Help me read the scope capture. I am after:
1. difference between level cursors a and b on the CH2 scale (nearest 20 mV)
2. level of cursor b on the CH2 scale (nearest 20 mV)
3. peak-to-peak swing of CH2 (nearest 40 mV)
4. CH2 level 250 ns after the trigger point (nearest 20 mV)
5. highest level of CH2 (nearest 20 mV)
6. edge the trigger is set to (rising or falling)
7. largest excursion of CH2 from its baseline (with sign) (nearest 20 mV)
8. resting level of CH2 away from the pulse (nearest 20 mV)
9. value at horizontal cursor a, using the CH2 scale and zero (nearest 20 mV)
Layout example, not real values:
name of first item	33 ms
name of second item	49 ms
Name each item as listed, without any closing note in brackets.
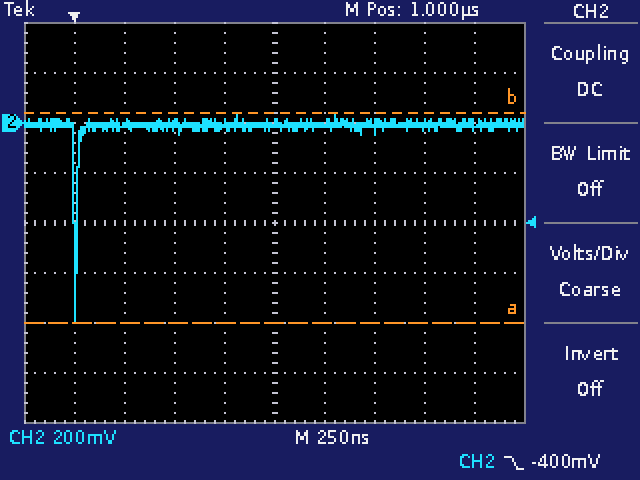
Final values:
difference between level cursors a and b on the CH2 scale	840 mV
level of cursor b on the CH2 scale	40 mV
peak-to-peak swing of CH2	840 mV
CH2 level 250 ns after the trigger point	0 mV
highest level of CH2	40 mV
edge the trigger is set to	falling
largest excursion of CH2 from its baseline (with sign)	-780 mV
resting level of CH2 away from the pulse	0 mV
value at horizontal cursor a, using the CH2 scale and zero	-800 mV
